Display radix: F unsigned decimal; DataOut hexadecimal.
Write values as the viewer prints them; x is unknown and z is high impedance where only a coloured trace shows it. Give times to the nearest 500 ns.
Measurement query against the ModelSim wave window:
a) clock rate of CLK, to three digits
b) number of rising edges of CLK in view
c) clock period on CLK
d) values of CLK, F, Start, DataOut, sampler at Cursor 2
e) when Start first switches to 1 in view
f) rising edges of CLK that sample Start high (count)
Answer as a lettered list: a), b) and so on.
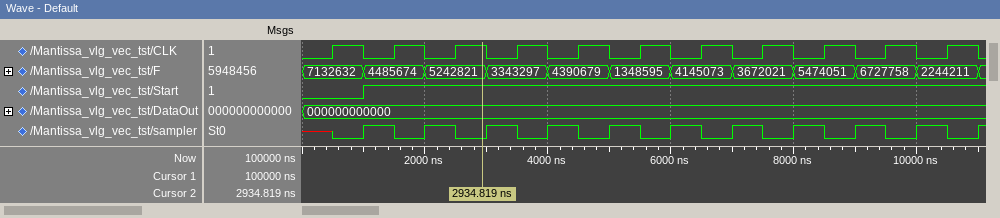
a) 1.00 MHz
b) 11
c) 1000 ns
d) CLK=1, F=5242821, Start=1, DataOut=000000000000, sampler=0
e) 1000 ns
f) 10
